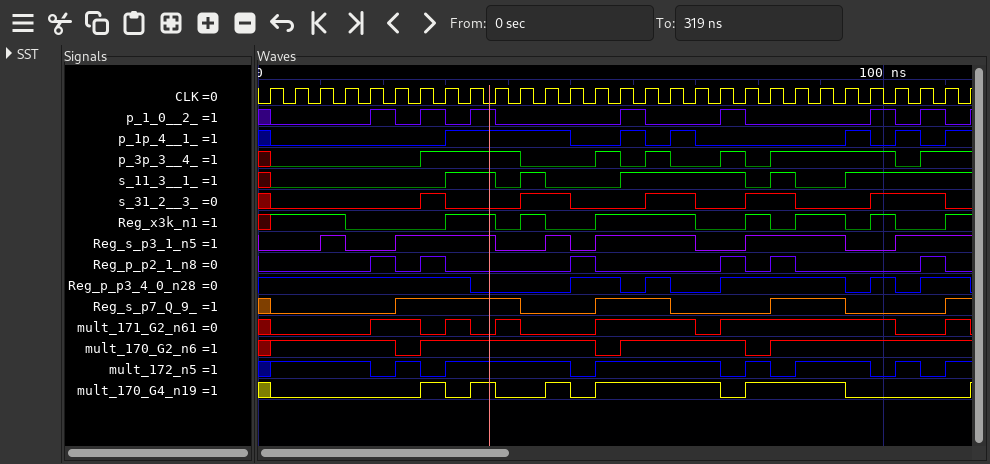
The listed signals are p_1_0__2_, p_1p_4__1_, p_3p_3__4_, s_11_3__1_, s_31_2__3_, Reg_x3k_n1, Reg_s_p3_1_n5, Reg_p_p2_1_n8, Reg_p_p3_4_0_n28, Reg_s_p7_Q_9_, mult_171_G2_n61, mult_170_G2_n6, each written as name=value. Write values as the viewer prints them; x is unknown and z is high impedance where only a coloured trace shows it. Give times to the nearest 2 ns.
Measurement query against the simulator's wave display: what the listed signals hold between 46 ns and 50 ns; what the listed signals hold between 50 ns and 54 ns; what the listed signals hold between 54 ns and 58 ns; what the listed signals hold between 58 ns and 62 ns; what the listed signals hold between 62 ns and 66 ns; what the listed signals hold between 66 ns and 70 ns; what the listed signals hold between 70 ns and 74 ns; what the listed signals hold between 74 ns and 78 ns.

p_1_0__2_=0, p_1p_4__1_=1, p_3p_3__4_=0, s_11_3__1_=0, s_31_2__3_=1, Reg_x3k_n1=0, Reg_s_p3_1_n5=1, Reg_p_p2_1_n8=0, Reg_p_p3_4_0_n28=0, Reg_s_p7_Q_9_=0, mult_171_G2_n61=0, mult_170_G2_n6=1
p_1_0__2_=0, p_1p_4__1_=0, p_3p_3__4_=0, s_11_3__1_=0, s_31_2__3_=0, Reg_x3k_n1=0, Reg_s_p3_1_n5=0, Reg_p_p2_1_n8=1, Reg_p_p3_4_0_n28=1, Reg_s_p7_Q_9_=0, mult_171_G2_n61=0, mult_170_G2_n6=1
p_1_0__2_=0, p_1p_4__1_=0, p_3p_3__4_=1, s_11_3__1_=0, s_31_2__3_=0, Reg_x3k_n1=1, Reg_s_p3_1_n5=1, Reg_p_p2_1_n8=0, Reg_p_p3_4_0_n28=1, Reg_s_p7_Q_9_=1, mult_171_G2_n61=1, mult_170_G2_n6=0
p_1_0__2_=1, p_1p_4__1_=1, p_3p_3__4_=0, s_11_3__1_=1, s_31_2__3_=0, Reg_x3k_n1=1, Reg_s_p3_1_n5=1, Reg_p_p2_1_n8=0, Reg_p_p3_4_0_n28=0, Reg_s_p7_Q_9_=1, mult_171_G2_n61=1, mult_170_G2_n6=1
p_1_0__2_=0, p_1p_4__1_=0, p_3p_3__4_=1, s_11_3__1_=1, s_31_2__3_=1, Reg_x3k_n1=1, Reg_s_p3_1_n5=1, Reg_p_p2_1_n8=0, Reg_p_p3_4_0_n28=1, Reg_s_p7_Q_9_=1, mult_171_G2_n61=1, mult_170_G2_n6=1
p_1_0__2_=0, p_1p_4__1_=1, p_3p_3__4_=0, s_11_3__1_=1, s_31_2__3_=1, Reg_x3k_n1=1, Reg_s_p3_1_n5=1, Reg_p_p2_1_n8=0, Reg_p_p3_4_0_n28=0, Reg_s_p7_Q_9_=0, mult_171_G2_n61=1, mult_170_G2_n6=1
p_1_0__2_=0, p_1p_4__1_=0, p_3p_3__4_=0, s_11_3__1_=1, s_31_2__3_=0, Reg_x3k_n1=0, Reg_s_p3_1_n5=0, Reg_p_p2_1_n8=0, Reg_p_p3_4_0_n28=0, Reg_s_p7_Q_9_=0, mult_171_G2_n61=0, mult_170_G2_n6=1
p_1_0__2_=1, p_1p_4__1_=0, p_3p_3__4_=1, s_11_3__1_=1, s_31_2__3_=0, Reg_x3k_n1=0, Reg_s_p3_1_n5=0, Reg_p_p2_1_n8=1, Reg_p_p3_4_0_n28=1, Reg_s_p7_Q_9_=0, mult_171_G2_n61=1, mult_170_G2_n6=1
